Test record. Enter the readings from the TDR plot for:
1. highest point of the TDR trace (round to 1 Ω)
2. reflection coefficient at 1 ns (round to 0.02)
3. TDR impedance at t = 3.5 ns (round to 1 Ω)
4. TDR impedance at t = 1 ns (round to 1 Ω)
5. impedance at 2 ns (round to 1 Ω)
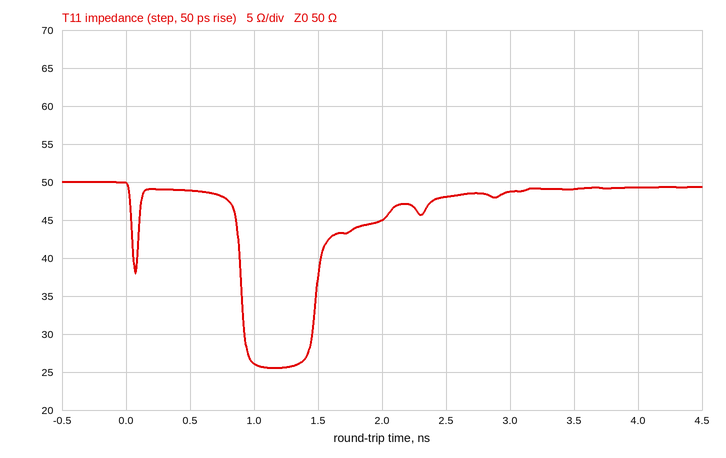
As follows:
50 Ω
-0.32
49 Ω
26 Ω
45 Ω
